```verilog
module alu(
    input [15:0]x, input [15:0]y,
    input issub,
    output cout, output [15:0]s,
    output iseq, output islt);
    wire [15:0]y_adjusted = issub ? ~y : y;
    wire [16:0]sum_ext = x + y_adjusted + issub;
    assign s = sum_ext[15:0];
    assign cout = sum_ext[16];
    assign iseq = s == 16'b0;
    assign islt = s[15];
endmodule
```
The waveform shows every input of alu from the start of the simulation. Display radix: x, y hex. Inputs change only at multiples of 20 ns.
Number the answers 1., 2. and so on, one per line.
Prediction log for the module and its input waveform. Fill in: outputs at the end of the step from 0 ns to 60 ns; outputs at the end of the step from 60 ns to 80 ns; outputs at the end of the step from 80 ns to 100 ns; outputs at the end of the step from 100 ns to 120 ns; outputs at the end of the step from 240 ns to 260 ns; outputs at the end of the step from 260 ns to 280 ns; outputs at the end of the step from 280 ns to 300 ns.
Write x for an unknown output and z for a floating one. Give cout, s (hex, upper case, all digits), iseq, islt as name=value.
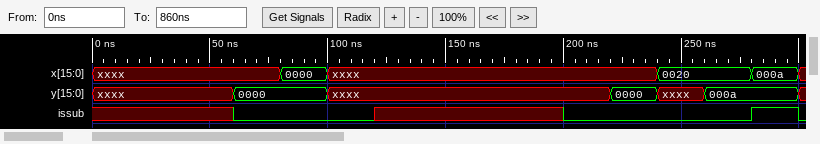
1. cout=x, s=x, iseq=x, islt=x
2. cout=x, s=x, iseq=x, islt=x
3. cout=0, s=0000, iseq=1, islt=0
4. cout=x, s=x, iseq=x, islt=x
5. cout=x, s=x, iseq=x, islt=x
6. cout=0, s=002A, iseq=0, islt=0
7. cout=1, s=0000, iseq=1, islt=0
